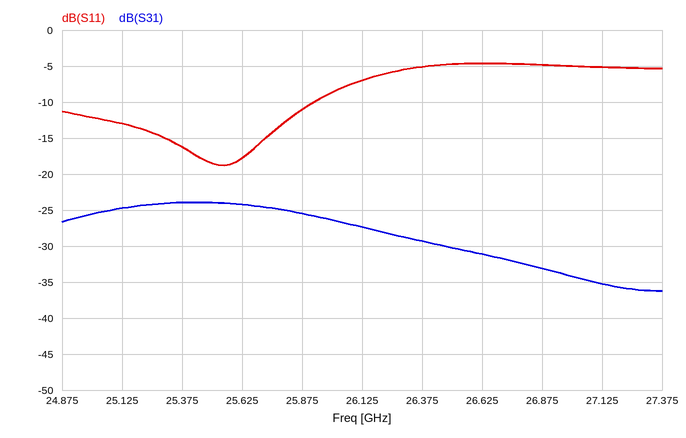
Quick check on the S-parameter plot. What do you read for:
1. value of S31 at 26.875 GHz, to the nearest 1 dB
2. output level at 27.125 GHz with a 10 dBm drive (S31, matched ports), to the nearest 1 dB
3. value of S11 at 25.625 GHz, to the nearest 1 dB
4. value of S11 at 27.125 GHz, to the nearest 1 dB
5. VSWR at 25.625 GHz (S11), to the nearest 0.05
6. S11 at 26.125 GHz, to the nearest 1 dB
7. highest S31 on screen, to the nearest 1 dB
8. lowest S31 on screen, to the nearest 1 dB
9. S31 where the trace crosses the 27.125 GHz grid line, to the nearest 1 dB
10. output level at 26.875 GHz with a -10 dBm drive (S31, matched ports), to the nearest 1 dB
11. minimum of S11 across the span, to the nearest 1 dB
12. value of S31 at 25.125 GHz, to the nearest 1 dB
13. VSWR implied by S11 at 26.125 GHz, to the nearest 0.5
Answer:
-33 dB
-25 dBm
-18 dB
-5 dB
1.30
-7 dB
-24 dB
-36 dB
-35 dB
-43 dBm
-19 dB
-25 dB
2.5
